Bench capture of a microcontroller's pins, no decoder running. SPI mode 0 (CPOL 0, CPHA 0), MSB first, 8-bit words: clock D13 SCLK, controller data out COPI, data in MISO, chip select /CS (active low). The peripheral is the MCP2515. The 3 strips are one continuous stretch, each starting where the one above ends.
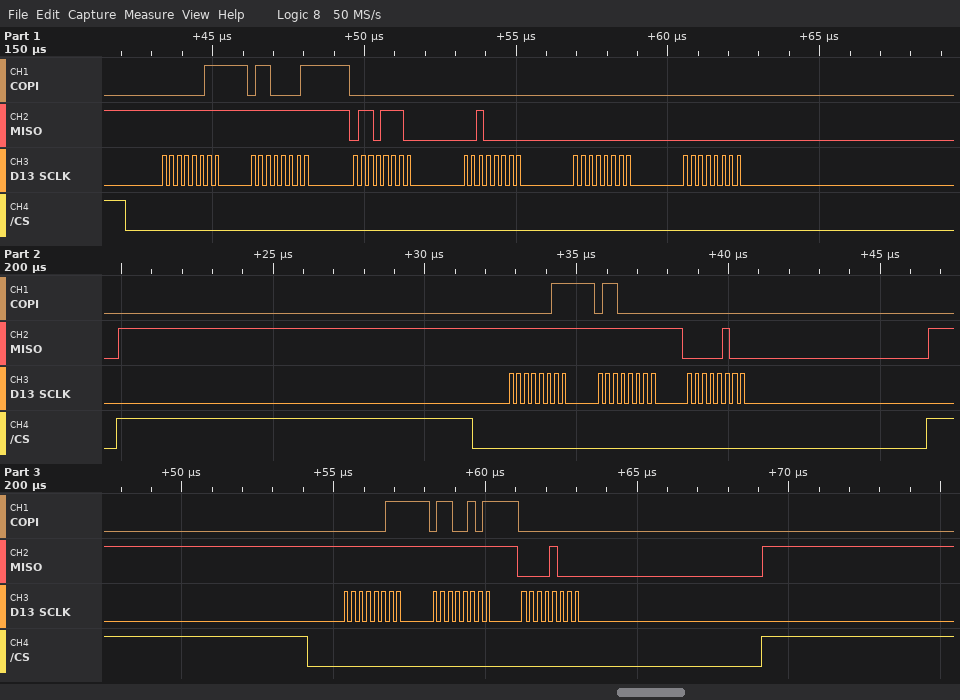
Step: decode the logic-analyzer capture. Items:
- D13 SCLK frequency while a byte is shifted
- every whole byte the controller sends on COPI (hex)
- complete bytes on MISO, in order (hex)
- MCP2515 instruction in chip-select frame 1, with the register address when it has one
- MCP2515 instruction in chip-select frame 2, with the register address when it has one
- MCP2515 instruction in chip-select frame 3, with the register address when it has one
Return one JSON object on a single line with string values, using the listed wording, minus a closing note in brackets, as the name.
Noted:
{"D13 SCLK frequency while a byte is shifted": "4 MHz", "every whole byte the controller sends on COPI": "03 61 00 00 00 00 03 60 00 03 65 00", "complete bytes on MISO, in order": "FF FF 6E 20 00 00 FF FF 04 FF FF 08", "MCP2515 instruction in chip-select frame 1, with the register address when it has one": "READ 0x61", "MCP2515 instruction in chip-select frame 2, with the register address when it has one": "READ 0x60", "MCP2515 instruction in chip-select frame 3, with the register address when it has one": "READ 0x65"}
